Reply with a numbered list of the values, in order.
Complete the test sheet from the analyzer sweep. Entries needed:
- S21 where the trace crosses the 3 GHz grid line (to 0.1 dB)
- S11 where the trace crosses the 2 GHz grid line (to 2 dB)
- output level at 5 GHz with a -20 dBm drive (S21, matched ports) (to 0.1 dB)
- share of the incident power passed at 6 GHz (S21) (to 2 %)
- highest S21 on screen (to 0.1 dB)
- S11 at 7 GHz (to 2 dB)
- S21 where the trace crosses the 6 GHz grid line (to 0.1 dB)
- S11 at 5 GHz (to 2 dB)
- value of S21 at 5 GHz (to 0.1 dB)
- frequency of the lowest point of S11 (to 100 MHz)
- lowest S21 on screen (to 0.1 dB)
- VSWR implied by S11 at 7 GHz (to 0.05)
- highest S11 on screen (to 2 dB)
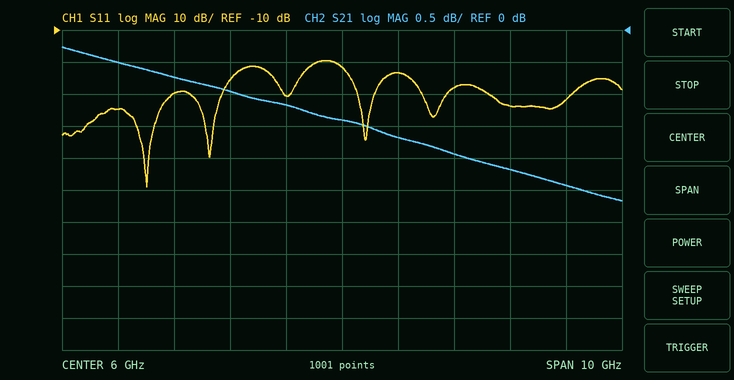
1. -0.7 dB
2. -34 dB
3. -21.2 dBm
4. 72 %
5. -0.3 dB
6. -24 dB
7. -1.4 dB
8. -30 dB
9. -1.2 dB
10. 2.5 GHz
11. -2.7 dB
12. 1.15
13. -20 dB
